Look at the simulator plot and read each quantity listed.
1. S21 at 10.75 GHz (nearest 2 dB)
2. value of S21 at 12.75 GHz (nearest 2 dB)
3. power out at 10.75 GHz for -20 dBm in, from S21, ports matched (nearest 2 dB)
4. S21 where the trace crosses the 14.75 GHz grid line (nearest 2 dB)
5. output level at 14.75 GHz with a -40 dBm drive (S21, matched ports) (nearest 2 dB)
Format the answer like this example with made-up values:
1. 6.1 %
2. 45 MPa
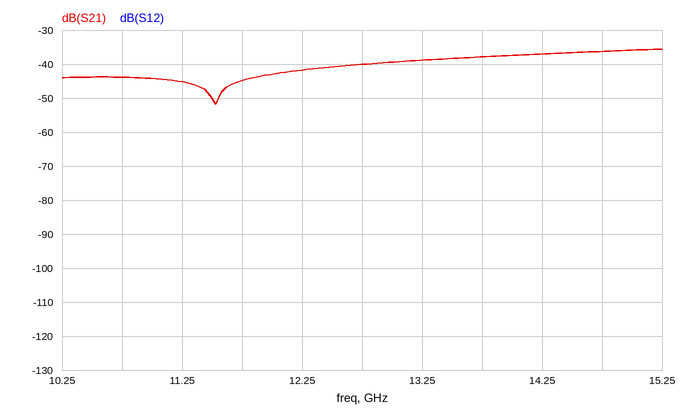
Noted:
1. -44 dB
2. -40 dB
3. -64 dBm
4. -36 dB
5. -76 dBm
